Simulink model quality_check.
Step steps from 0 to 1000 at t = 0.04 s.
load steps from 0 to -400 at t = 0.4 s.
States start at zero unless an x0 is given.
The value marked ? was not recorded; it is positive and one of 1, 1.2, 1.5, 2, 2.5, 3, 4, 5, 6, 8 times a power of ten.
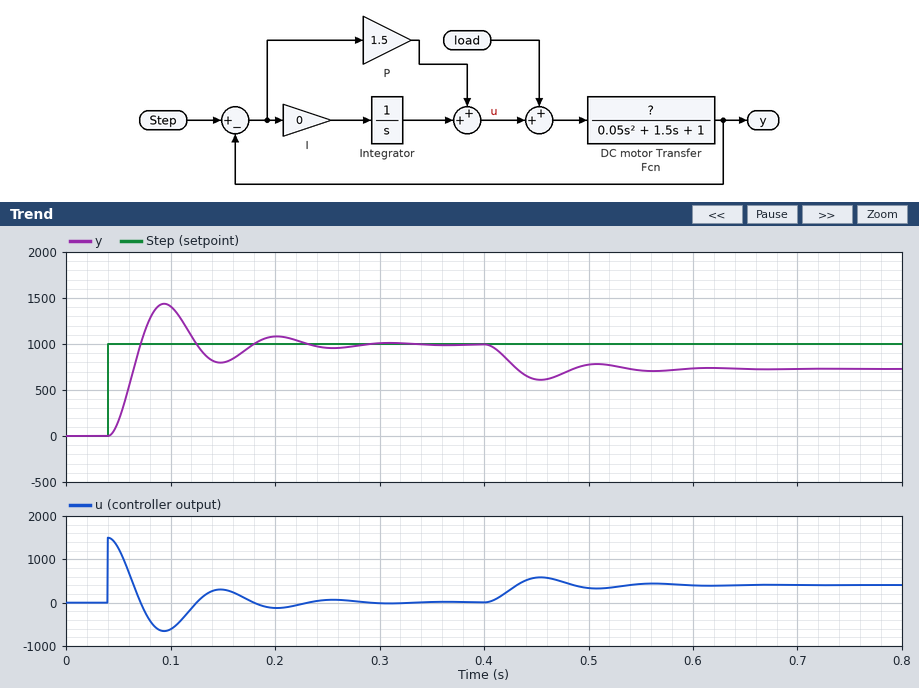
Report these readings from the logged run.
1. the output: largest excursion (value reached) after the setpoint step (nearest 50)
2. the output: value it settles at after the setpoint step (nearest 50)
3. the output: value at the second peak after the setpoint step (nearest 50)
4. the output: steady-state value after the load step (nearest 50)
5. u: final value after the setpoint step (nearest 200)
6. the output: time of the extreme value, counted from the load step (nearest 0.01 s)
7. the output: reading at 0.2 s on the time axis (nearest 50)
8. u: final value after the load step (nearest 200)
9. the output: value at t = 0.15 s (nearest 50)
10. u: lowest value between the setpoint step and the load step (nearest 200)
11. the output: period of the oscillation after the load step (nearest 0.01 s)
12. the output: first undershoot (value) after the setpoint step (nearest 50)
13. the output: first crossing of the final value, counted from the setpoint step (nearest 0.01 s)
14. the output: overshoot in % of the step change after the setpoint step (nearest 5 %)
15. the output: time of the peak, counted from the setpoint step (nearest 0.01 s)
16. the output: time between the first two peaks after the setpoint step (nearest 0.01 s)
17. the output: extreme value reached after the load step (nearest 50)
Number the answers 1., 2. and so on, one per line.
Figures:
1. 1450
2. 1000
3. 1100
4. 750
5. 0
6. 0.05 s
7. 1100
8. 400
9. 800
10. -600
11. 0.11 s
12. 800
13. 0.03 s
14. 45 %
15. 0.05 s
16. 0.11 s
17. 600
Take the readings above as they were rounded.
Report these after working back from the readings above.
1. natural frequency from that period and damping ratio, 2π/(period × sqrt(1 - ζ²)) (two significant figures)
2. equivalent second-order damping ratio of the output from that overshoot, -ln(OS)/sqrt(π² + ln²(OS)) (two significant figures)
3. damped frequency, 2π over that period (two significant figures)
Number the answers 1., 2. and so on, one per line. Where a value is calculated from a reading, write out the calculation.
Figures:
1. 2π / (0.11 × sqrt(1 - 0.25²)) = 59 rad/s
2. ln(0.45) = -0.799; 0.799 / sqrt(9.870 + 0.638) = 0.25
3. 2π / 0.11 = 57 rad/s
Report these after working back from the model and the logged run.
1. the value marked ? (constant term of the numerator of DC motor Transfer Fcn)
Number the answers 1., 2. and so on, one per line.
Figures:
1. 120
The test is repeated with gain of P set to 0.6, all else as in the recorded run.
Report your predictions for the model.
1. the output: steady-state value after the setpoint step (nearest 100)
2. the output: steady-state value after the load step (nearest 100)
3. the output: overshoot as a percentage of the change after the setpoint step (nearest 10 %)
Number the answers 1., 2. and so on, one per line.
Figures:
1. 1000
2. 300
3. 30 %
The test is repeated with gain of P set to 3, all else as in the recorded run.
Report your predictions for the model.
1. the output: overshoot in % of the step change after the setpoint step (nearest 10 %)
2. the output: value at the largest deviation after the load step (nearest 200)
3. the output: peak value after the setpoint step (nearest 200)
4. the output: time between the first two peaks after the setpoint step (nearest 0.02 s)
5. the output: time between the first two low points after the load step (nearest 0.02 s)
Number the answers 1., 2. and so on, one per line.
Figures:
1. 60 %
2. 800
3. 1600
4. 0.08 s
5. 0.08 s
